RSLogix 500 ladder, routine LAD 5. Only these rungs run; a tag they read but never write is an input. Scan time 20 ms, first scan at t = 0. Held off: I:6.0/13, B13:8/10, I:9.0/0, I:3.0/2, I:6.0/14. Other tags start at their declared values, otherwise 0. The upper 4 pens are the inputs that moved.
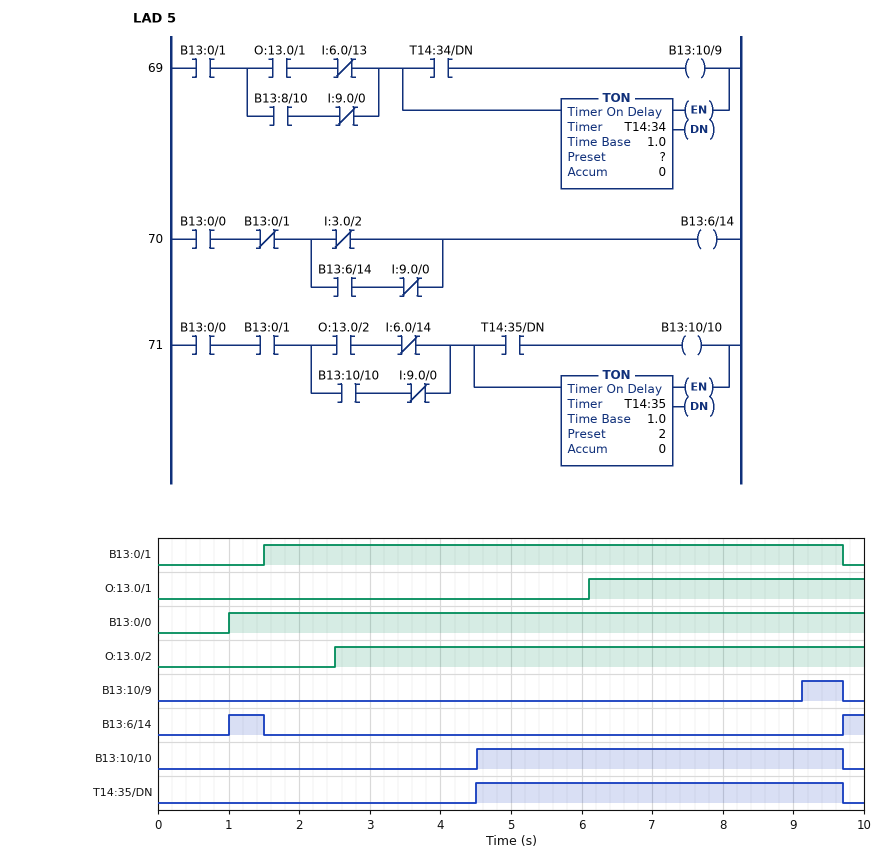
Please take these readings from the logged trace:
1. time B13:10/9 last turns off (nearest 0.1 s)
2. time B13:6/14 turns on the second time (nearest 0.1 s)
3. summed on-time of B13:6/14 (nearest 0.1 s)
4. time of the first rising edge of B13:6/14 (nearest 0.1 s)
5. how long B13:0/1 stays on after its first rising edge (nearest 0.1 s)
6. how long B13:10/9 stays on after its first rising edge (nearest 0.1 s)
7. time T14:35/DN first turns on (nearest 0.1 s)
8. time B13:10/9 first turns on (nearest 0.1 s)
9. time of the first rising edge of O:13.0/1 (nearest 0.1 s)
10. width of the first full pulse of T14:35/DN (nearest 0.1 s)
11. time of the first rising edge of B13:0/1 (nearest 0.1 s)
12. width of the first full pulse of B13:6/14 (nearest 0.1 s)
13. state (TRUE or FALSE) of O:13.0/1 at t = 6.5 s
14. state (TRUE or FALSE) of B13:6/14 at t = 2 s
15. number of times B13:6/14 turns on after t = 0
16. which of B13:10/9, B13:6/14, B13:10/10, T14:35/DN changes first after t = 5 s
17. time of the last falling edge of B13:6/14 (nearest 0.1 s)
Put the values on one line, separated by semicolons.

9.7 s; 9.7 s; 0.8 s; 1.0 s; 8.2 s; 0.6 s; 4.5 s; 9.1 s; 6.1 s; 5.2 s; 1.5 s; 0.5 s; TRUE; FALSE; 2; B13:10/9; 1.5 s
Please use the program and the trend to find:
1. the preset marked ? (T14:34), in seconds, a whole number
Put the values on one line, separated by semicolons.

3 s
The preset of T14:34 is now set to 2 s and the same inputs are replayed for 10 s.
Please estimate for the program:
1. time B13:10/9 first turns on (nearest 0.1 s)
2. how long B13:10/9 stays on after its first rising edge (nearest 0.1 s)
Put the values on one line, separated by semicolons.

8.1 s; 1.6 s
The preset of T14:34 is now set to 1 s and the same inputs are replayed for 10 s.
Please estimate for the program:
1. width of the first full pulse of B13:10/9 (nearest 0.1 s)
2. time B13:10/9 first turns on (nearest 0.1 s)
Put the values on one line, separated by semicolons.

2.6 s; 7.1 s
